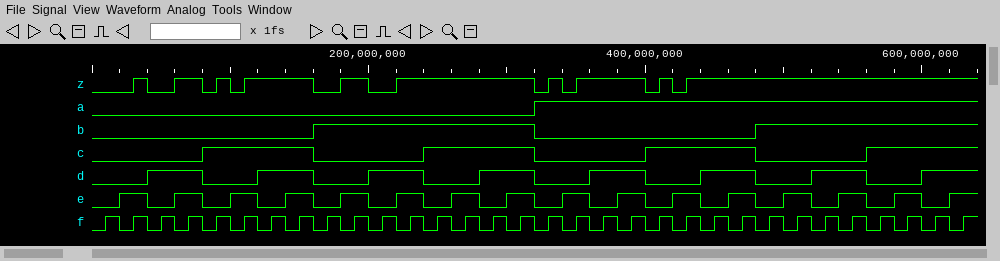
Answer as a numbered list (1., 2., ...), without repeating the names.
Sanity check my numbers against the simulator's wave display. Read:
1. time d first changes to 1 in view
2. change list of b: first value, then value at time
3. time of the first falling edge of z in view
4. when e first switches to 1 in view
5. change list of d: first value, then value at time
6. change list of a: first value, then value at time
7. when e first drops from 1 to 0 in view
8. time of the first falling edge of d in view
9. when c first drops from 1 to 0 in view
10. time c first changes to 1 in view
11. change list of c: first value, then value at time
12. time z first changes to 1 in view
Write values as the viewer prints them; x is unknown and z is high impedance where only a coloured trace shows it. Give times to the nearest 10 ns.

1. 40 ns
2. 0, 1 at 160 ns, 0 at 320 ns, 1 at 480 ns
3. 40 ns
4. 20 ns
5. 0, 1 at 40 ns, 0 at 80 ns, 1 at 120 ns, 0 at 160 ns, 1 at 200 ns, 0 at 240 ns, 1 at 280 ns, 0 at 320 ns, 1 at 360 ns, 0 at 400 ns, 1 at 440 ns, 0 at 480 ns, 1 at 520 ns, 0 at 560 ns, 1 at 600 ns
6. 0, 1 at 320 ns
7. 40 ns
8. 80 ns
9. 160 ns
10. 80 ns
11. 0, 1 at 80 ns, 0 at 160 ns, 1 at 240 ns, 0 at 320 ns, 1 at 400 ns, 0 at 480 ns, 1 at 560 ns
12. 30 ns
